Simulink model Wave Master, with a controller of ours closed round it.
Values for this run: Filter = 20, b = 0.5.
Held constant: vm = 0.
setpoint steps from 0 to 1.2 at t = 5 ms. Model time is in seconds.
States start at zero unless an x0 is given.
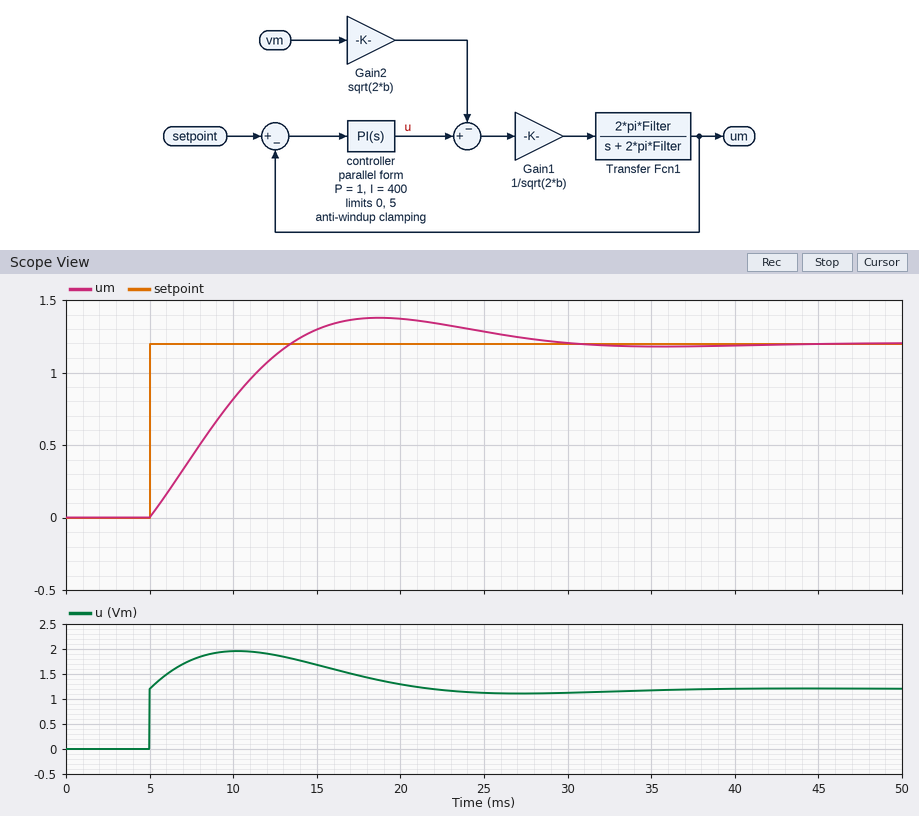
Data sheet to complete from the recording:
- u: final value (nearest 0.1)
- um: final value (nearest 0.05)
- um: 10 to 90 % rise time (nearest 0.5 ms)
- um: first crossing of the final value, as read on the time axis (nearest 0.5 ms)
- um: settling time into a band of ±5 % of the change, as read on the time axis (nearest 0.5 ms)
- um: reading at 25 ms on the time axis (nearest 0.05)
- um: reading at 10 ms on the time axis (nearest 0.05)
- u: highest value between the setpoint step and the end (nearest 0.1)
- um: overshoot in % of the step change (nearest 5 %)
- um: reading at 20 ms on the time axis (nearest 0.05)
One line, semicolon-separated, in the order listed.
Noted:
1.2; 1.20; 6.5 ms; 13.5 ms; 26.0 ms; 1.30; 0.80; 2.0; 15 %; 1.35
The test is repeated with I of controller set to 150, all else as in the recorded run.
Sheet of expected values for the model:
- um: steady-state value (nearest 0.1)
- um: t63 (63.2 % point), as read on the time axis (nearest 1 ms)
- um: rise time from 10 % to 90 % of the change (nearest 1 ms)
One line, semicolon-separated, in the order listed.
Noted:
1.2; 12 ms; 14 ms
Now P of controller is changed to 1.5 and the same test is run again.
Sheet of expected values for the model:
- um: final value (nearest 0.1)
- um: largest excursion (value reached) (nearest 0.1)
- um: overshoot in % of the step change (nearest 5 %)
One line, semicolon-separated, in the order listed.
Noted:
1.2; 1.3; 10 %
